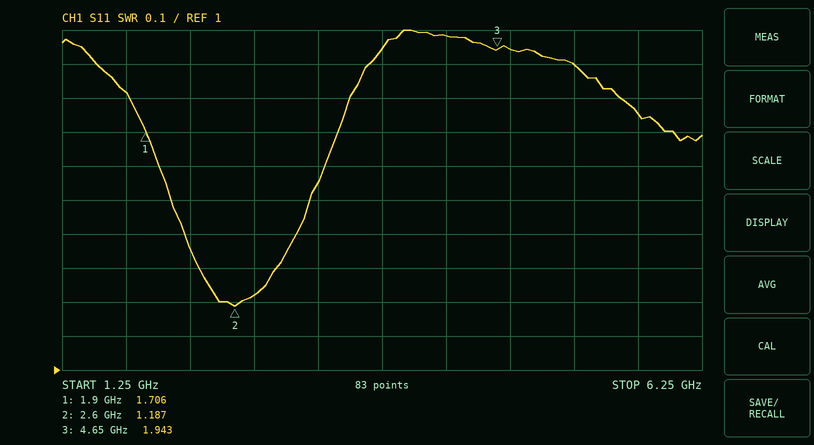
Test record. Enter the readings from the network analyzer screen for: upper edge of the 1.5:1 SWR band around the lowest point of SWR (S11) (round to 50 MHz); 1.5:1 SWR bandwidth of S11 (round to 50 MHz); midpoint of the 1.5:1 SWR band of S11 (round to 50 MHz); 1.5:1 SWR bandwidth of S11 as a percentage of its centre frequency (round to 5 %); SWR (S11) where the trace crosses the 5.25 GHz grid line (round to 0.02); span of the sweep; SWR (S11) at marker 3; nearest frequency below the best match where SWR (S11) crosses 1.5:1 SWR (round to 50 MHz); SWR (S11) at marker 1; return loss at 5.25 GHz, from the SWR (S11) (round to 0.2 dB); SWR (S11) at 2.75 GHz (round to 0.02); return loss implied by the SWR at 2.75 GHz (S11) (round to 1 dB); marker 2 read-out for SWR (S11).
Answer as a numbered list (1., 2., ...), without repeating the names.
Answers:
1. 3.20 GHz
2. 1.10 GHz
3. 2.65 GHz
4. 40 %
5. 1.90
6. 5 GHz
7. 1.943
8. 2.10 GHz
9. 1.706
10. 10.2 dB
11. 1.22
12. 20 dB
13. 1.187
